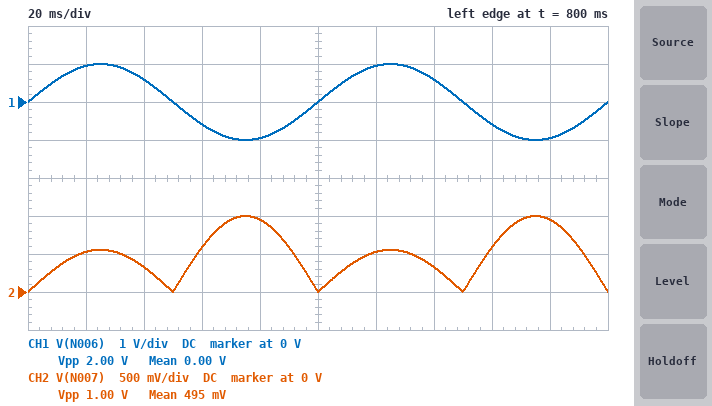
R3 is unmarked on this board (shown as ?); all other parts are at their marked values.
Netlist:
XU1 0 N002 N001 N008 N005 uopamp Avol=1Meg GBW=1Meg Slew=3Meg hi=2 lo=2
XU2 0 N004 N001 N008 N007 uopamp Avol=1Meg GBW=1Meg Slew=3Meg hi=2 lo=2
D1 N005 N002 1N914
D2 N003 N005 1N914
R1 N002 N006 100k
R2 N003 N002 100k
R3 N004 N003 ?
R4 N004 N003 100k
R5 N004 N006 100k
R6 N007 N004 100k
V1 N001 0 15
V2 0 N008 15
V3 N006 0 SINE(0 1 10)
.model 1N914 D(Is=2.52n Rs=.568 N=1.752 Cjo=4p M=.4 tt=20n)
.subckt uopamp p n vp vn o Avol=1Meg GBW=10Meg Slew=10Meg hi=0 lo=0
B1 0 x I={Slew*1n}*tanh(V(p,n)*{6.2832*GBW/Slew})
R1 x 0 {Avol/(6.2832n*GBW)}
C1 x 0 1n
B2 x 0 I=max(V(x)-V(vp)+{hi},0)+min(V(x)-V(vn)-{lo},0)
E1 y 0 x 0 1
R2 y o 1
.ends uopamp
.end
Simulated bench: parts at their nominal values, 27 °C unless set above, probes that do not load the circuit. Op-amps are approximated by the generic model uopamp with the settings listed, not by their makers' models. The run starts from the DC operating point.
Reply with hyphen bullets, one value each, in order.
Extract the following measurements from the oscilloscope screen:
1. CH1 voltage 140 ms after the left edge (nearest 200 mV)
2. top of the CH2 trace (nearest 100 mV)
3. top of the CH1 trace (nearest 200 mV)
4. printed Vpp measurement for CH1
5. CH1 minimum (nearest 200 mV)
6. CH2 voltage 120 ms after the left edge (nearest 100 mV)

- 600 mV
- 1.0 V
- 1.0 V
- 2.00 V
- -1.0 V
- 500 mV
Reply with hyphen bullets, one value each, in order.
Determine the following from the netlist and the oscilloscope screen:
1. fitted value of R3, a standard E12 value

- 180 kΩ
